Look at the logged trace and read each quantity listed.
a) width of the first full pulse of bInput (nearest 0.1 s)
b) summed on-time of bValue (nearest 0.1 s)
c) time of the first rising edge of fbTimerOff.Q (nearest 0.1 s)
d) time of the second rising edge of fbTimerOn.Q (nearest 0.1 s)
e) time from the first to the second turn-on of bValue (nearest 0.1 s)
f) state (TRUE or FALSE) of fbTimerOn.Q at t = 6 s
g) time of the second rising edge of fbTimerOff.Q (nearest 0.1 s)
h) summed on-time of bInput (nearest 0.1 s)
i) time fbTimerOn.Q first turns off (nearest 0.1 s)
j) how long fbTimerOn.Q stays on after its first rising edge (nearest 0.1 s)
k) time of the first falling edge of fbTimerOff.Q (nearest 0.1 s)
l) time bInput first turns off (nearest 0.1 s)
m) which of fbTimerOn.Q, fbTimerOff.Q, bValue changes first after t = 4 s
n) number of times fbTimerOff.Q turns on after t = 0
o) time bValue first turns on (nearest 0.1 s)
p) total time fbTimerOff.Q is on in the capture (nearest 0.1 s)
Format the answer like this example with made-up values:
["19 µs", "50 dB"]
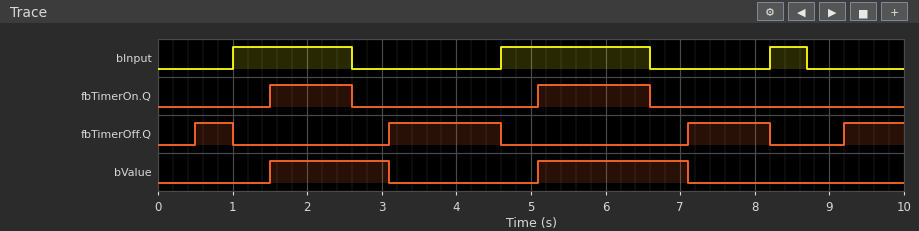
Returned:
["1.6 s", "3.6 s", "0.5 s", "5.1 s", "3.6 s", "TRUE", "3.1 s", "4.1 s", "2.6 s", "1.1 s", "1.0 s", "2.6 s", "fbTimerOff.Q", "4", "1.5 s", "3.9 s"]
